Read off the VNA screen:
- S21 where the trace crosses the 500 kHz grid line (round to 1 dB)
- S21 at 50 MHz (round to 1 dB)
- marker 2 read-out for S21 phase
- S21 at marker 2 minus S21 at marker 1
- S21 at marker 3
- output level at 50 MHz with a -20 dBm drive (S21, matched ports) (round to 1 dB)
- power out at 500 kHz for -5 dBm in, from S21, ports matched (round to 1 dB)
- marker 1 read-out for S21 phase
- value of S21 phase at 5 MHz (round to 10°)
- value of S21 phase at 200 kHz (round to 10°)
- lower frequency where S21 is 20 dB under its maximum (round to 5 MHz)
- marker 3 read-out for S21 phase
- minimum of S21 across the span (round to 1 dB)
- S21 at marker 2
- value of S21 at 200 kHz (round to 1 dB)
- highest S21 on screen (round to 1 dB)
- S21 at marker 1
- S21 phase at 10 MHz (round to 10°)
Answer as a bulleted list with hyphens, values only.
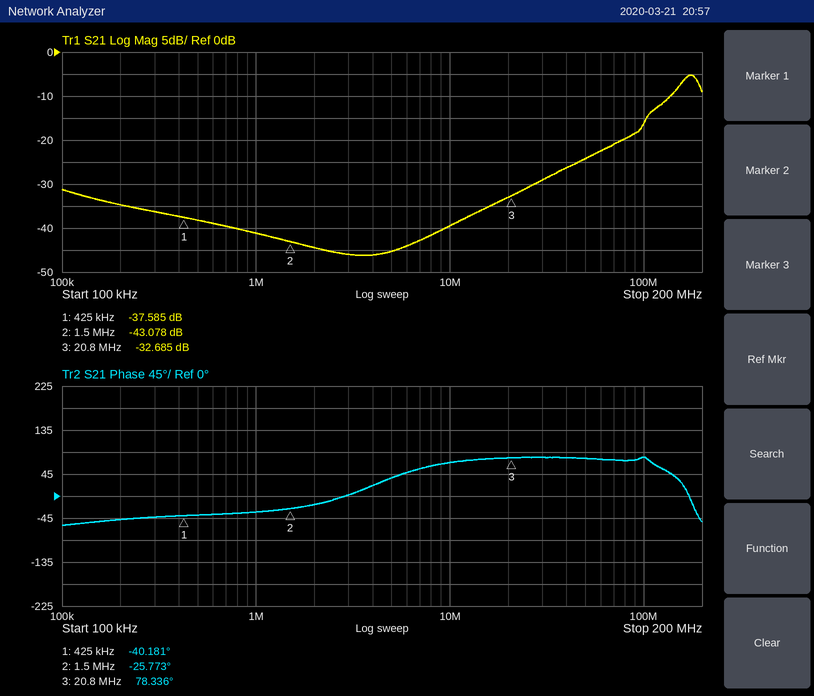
- -38 dB
- -24 dB
- -25.773°
- -5.493 dB
- -32.685 dB
- -44 dBm
- -43 dBm
- -40.181°
- 40°
- -50°
- 45 MHz
- 78.336°
- -46 dB
- -43.078 dB
- -35 dB
- -5 dB
- -37.585 dB
- 70°
